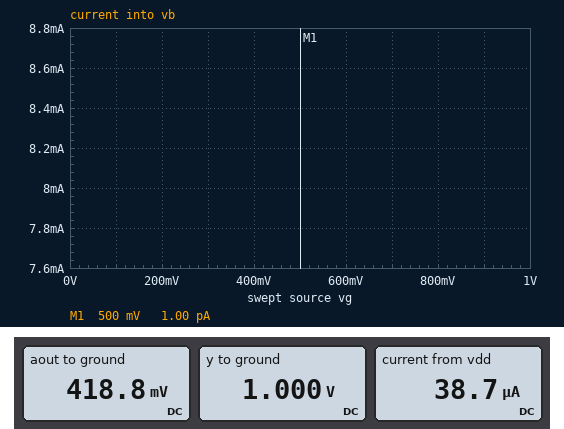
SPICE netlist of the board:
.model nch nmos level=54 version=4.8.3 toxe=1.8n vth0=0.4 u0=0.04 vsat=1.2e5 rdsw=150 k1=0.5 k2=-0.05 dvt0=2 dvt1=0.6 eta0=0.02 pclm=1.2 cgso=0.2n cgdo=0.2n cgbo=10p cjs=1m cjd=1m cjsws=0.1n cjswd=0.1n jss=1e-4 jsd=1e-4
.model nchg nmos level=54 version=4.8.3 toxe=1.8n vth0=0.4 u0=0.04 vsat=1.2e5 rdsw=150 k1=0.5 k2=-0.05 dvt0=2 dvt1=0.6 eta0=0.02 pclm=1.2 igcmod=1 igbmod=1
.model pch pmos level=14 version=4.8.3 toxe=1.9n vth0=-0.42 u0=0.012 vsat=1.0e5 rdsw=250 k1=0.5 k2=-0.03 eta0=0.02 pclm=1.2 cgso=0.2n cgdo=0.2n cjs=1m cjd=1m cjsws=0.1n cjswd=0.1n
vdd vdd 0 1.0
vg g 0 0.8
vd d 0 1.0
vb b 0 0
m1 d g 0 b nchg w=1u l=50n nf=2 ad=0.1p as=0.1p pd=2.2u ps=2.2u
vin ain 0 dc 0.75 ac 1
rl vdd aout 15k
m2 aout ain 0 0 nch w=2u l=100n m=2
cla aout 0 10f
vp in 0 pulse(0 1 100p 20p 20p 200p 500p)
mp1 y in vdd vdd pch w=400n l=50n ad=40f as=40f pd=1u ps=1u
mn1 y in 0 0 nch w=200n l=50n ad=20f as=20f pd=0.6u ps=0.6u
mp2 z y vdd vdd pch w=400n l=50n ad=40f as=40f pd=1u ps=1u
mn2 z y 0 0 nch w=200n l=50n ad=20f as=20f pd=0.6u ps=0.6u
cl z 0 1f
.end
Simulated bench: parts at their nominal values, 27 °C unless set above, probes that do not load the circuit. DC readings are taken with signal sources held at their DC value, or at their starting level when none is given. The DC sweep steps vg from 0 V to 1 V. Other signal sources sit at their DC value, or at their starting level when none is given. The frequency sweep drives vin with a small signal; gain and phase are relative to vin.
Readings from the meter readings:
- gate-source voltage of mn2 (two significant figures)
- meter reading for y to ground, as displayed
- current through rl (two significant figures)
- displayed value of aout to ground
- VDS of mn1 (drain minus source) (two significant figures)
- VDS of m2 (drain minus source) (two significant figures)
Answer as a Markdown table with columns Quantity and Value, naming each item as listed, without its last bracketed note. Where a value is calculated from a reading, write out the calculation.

| Quantity | Value |
|---|---|
| gate-source voltage of mn2 | 1 V = 1.0 V |
| meter reading for y to ground, as displayed | 1.000 V |
| current through rl | (1 V - 418.8 mV) / 15 kΩ = 39 µA |
| displayed value of aout to ground | 418.8 mV |
| VDS of mn1 (drain minus source) | 1 V = 1.0 V |
| VDS of m2 (drain minus source) | 418.8 mV = 420 mV |
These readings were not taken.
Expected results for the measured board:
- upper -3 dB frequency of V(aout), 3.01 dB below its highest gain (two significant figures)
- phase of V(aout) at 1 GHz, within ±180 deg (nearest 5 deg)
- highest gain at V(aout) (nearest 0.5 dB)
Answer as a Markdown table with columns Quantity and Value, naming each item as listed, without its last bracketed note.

| Quantity | Value |
|---|---|
| upper -3 dB frequency of V(aout), 3.01 dB below its highest gain | 1.4 GHz |
| phase of V(aout) at 1 GHz, within ±180 deg | 145 deg |
| highest gain at V(aout) | 18.0 dB |
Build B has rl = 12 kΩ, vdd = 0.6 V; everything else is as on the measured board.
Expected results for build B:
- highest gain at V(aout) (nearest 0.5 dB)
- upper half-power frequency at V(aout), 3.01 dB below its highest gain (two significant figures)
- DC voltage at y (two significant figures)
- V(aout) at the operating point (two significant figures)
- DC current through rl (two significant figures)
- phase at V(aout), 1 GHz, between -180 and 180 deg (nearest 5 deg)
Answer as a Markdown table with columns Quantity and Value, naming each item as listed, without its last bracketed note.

| Quantity | Value |
|---|---|
| highest gain at V(aout) | 15.0 dB |
| upper half-power frequency at V(aout), 3.01 dB below its highest gain | 1.7 GHz |
| DC voltage at y | 600 mV |
| V(aout) at the operating point | 230 mV |
| DC current through rl | 31 µA |
| phase at V(aout), 1 GHz, between -180 and 180 deg | 150 deg |
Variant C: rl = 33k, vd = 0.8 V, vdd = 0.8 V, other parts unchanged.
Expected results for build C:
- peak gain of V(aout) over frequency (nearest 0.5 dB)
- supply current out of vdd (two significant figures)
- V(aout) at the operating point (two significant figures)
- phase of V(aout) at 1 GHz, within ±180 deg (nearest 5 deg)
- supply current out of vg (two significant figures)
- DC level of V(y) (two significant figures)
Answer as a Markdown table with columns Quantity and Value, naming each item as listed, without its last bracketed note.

| Quantity | Value |
|---|---|
| peak gain of V(aout) over frequency | 10.5 dB |
| supply current out of vdd | 22 µA |
| V(aout) at the operating point | 74 mV |
| phase of V(aout) at 1 GHz, within ±180 deg | 150 deg |
| supply current out of vg | 280 mA |
| DC level of V(y) | 800 mV |
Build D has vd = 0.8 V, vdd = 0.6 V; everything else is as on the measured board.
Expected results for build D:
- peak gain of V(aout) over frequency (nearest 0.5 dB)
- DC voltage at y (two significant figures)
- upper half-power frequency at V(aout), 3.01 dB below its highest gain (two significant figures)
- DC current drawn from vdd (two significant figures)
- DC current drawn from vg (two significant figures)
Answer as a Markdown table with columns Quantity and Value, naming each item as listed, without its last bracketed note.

| Quantity | Value |
|---|---|
| peak gain of V(aout) over frequency | 15.5 dB |
| DC voltage at y | 600 mV |
| upper half-power frequency at V(aout), 3.01 dB below its highest gain | 1.5 GHz |
| DC current drawn from vdd | 28 µA |
| DC current drawn from vg | 280 mA |
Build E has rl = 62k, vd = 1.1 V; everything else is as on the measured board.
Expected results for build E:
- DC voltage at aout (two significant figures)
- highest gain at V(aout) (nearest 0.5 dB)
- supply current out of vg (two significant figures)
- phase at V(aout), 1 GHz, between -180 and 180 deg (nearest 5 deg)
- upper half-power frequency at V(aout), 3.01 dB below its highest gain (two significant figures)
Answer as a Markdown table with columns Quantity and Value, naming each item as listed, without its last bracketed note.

| Quantity | Value |
|---|---|
| DC voltage at aout | 39 mV |
| highest gain at V(aout) | 1.0 dB |
| supply current out of vg | 350 mA |
| phase at V(aout), 1 GHz, between -180 and 180 deg | 160 deg |
| upper half-power frequency at V(aout), 3.01 dB below its highest gain | 3.8 GHz |
